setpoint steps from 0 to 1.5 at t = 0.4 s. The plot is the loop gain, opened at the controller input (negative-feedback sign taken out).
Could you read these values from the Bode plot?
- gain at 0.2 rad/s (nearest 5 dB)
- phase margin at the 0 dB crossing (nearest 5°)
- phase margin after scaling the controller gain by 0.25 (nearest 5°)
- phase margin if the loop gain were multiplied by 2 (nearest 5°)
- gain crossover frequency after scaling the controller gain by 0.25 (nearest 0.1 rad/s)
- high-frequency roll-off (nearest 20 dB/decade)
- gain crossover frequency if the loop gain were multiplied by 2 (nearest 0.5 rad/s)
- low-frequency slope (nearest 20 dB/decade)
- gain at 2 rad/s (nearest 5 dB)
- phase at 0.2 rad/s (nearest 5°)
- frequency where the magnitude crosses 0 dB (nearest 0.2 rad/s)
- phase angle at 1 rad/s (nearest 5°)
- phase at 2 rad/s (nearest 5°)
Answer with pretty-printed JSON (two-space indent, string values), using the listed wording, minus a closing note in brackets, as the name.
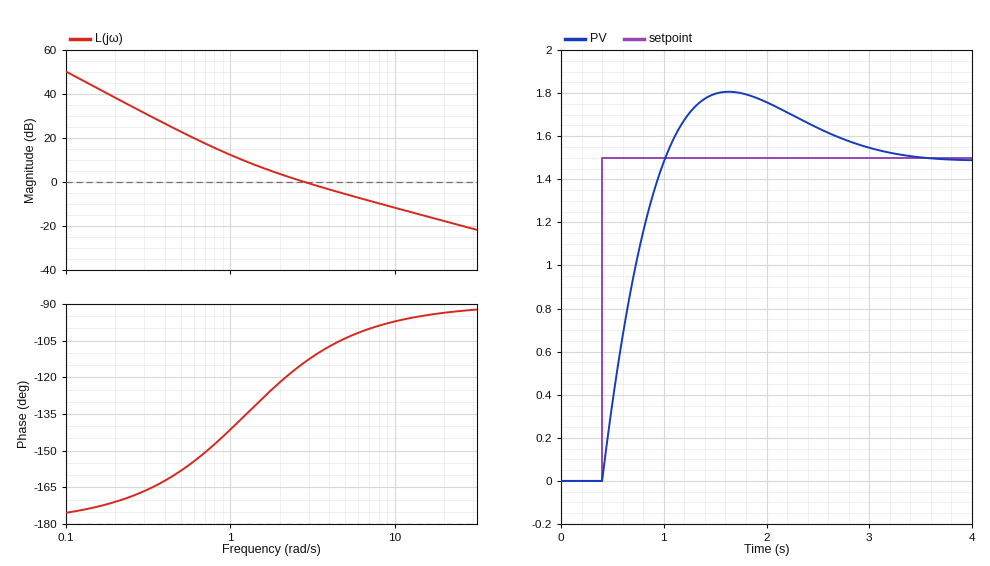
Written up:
{
  "gain at 0.2 rad/s": "40 dB",
  "phase margin at the 0 dB crossing": "65°",
  "phase margin after scaling the controller gain by 0.25": "40°",
  "phase margin if the loop gain were multiplied by 2": "75°",
  "gain crossover frequency after scaling the controller gain by 0.25": "1.0 rad/s",
  "high-frequency roll-off": "-20 dB/decade",
  "gain crossover frequency if the loop gain were multiplied by 2": "5.5 rad/s",
  "low-frequency slope": "-40 dB/decade",
  "gain at 2 rad/s": "5 dB",
  "phase at 0.2 rad/s": "-170°",
  "frequency where the magnitude crosses 0 dB": "2.8 rad/s",
  "phase angle at 1 rad/s": "-140°",
  "phase at 2 rad/s": "-120°"
}
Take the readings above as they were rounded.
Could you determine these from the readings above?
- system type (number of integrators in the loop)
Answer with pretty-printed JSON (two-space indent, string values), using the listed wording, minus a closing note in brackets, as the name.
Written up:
{
  "system type": "2"
}
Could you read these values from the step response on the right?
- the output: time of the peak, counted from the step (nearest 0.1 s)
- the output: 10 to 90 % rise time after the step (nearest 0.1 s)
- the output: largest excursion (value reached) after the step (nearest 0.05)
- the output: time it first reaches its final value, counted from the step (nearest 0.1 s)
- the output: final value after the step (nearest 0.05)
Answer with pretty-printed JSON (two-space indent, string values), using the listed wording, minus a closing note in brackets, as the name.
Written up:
{
  "the output: time of the peak, counted from the step": "1.2 s",
  "the output: 10 to 90 % rise time after the step": "0.5 s",
  "the output: largest excursion (value reached) after the step": "1.80",
  "the output: time it first reaches its final value, counted from the step": "0.6 s",
  "the output: final value after the step": "1.50"
}
